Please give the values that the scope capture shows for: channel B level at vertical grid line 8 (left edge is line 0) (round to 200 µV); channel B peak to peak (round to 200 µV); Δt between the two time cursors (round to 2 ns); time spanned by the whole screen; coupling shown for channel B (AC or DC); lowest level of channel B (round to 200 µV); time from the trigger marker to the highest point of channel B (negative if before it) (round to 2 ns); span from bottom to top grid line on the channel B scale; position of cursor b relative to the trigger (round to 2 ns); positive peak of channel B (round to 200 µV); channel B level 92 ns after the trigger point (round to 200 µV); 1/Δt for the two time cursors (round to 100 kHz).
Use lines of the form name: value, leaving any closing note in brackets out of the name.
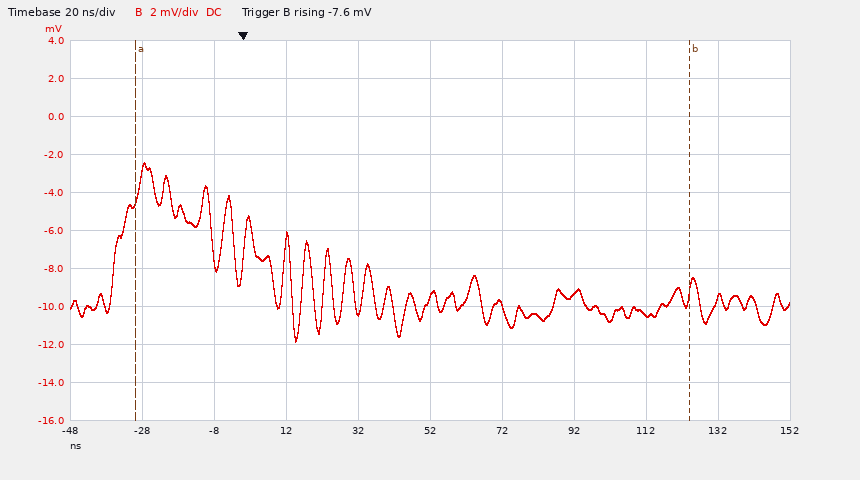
channel B level at vertical grid line 8 (left edge is line 0): -10.4 mV
channel B peak to peak: 9.4 mV
Δt between the two time cursors: 154 ns
time spanned by the whole screen: 200 ns
coupling shown for channel B: DC
lowest level of channel B: -11.8 mV
time from the trigger marker to the highest point of channel B (negative if before it): -28 ns
span from bottom to top grid line on the channel B scale: 20 mV
position of cursor b relative to the trigger: +124 ns
positive peak of channel B: -2.4 mV
channel B level 92 ns after the trigger point: -9.4 mV
1/Δt for the two time cursors: 6.5 MHz
